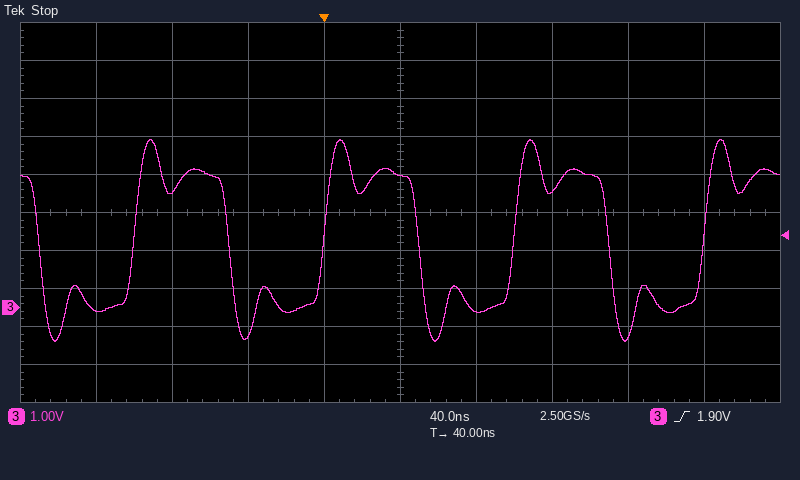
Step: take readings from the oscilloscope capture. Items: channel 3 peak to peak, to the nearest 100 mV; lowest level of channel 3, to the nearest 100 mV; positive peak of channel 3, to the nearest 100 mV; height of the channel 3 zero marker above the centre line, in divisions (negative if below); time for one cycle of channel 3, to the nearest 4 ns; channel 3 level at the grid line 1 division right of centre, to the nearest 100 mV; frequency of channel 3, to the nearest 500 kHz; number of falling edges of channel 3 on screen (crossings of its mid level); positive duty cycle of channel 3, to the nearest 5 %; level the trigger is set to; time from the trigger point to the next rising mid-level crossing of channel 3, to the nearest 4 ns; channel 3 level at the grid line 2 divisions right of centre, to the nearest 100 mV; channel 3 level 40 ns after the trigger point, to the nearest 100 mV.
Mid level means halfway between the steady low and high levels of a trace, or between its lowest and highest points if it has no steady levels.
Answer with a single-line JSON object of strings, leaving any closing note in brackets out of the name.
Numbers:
{"channel 3 peak to peak, to the nearest 100 mV": "5.3 V", "lowest level of channel 3, to the nearest 100 mV": "-900 mV", "positive peak of channel 3, to the nearest 100 mV": "4.4 V", "height of the channel 3 zero marker above the centre line, in divisions": "-2.5 div", "time for one cycle of channel 3, to the nearest 4 ns": "100 ns", "channel 3 level at the grid line 1 division right of centre, to the nearest 100 mV": "-100 mV", "frequency of channel 3, to the nearest 500 kHz": "10.0 MHz", "number of falling edges of channel 3 on screen": "4", "positive duty cycle of channel 3, to the nearest 5 %": "50 %", "level the trigger is set to": "1.90 V", "time from the trigger point to the next rising mid-level crossing of channel 3, to the nearest 4 ns": "100 ns", "channel 3 level at the grid line 2 divisions right of centre, to the nearest 100 mV": "3.1 V", "channel 3 level 40 ns after the trigger point, to the nearest 100 mV": "3.5 V"}
